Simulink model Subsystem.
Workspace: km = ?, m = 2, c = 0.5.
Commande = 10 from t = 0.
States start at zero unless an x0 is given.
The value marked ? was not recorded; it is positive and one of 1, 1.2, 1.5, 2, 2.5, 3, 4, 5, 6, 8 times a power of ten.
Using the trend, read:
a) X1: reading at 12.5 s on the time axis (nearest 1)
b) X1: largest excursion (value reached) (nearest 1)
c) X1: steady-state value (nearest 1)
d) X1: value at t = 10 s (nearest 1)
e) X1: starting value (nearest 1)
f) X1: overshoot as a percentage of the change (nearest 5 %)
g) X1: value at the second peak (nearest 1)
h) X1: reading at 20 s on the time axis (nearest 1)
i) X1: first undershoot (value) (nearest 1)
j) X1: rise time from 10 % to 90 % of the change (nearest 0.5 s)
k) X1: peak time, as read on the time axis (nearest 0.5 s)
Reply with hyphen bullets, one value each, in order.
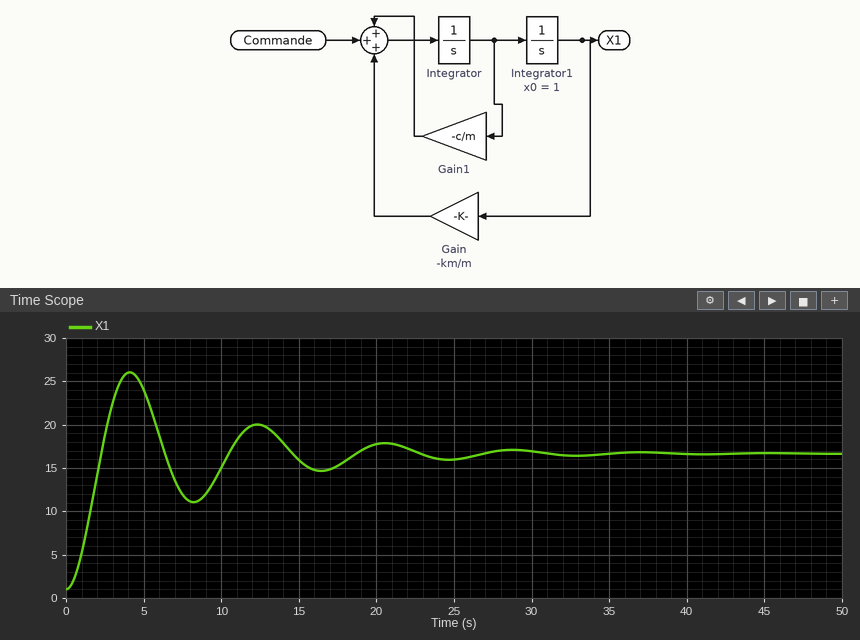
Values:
- 20
- 26
- 17
- 15
- 1
- 60 %
- 20
- 18
- 11
- 1.5 s
- 4.0 s
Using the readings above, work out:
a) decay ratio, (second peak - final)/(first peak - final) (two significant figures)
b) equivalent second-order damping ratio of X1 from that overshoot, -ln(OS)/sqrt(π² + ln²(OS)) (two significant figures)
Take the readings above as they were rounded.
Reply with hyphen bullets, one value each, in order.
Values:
- 0.33
- 0.16
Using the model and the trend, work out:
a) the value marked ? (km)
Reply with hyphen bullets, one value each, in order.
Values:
- 1.2
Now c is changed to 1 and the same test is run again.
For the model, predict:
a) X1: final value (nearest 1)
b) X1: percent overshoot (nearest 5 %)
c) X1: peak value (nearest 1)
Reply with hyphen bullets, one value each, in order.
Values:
- 17
- 35 %
- 22
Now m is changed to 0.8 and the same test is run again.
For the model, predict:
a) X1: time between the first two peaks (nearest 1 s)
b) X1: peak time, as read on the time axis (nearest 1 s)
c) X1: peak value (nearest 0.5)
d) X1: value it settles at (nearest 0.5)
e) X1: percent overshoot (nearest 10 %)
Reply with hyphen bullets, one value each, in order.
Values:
- 5 s
- 3 s
- 9.0
- 6.5
- 40 %
